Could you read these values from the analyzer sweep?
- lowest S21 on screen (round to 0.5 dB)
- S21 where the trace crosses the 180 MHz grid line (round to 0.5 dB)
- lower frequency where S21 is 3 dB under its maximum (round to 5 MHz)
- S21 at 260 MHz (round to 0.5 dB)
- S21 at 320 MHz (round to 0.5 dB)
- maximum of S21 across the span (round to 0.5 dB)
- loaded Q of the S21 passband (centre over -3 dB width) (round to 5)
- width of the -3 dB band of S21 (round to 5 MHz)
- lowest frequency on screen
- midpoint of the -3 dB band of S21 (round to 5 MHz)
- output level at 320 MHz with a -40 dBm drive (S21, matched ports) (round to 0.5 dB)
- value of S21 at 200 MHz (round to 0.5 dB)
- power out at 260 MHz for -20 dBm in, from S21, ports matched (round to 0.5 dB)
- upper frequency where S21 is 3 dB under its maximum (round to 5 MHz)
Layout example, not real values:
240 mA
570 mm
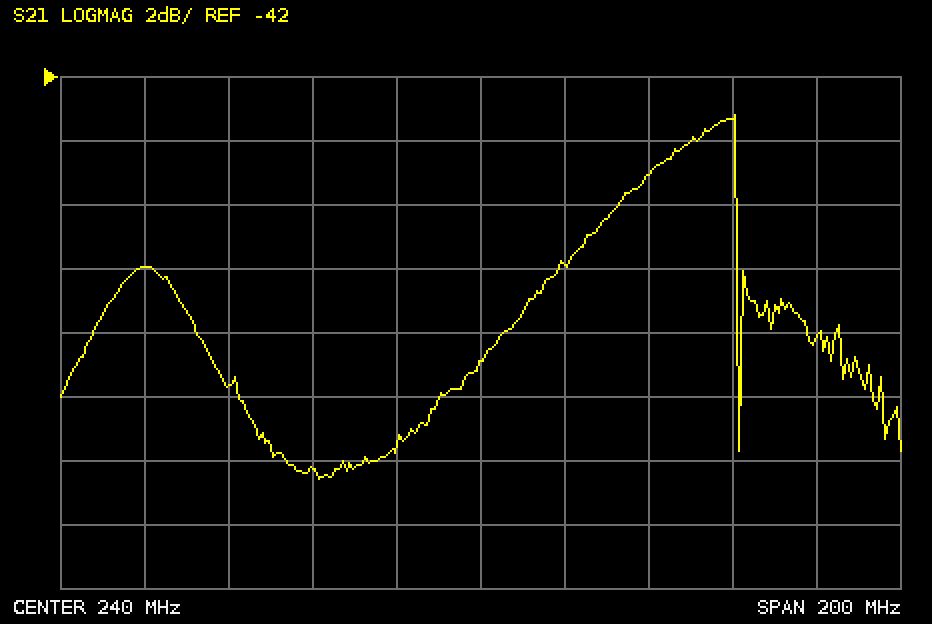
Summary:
-54.5 dB
-51.5 dB
270 MHz
-48.0 dB
-50.0 dB
-43.0 dB
10
30 MHz
140 MHz
285 MHz
-90.0 dBm
-54.0 dB
-68.0 dBm
300 MHz
